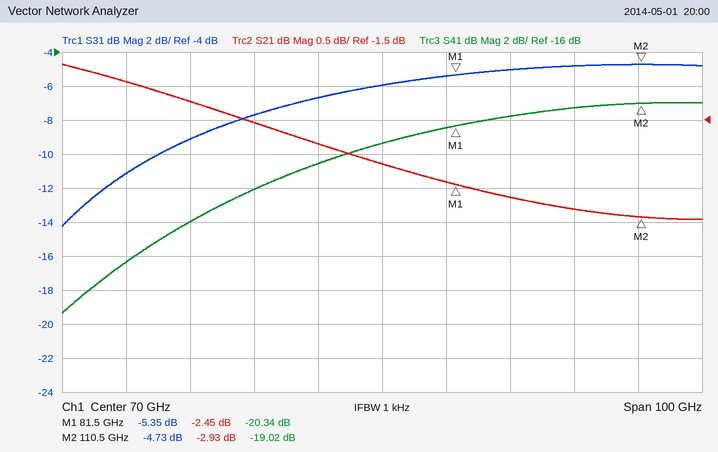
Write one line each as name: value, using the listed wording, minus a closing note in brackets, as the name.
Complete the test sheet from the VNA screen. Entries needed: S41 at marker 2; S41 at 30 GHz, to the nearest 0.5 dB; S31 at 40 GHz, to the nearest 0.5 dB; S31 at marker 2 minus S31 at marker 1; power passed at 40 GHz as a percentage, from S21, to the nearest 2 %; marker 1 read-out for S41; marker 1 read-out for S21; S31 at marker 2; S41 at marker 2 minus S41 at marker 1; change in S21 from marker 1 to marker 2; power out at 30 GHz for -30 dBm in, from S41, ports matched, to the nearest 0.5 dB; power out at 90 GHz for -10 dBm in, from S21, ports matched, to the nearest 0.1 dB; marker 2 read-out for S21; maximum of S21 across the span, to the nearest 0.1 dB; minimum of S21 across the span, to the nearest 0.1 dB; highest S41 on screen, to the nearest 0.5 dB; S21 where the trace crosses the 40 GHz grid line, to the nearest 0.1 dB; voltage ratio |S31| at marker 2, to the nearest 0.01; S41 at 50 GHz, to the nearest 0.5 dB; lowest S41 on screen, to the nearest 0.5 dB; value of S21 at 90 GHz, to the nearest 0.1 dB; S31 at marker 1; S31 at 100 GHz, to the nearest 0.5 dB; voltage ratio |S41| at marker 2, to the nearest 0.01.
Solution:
S41 at marker 2: -19.02 dB
S41 at 30 GHz, to the nearest 0.5 dB: -28.5 dB
S31 at 40 GHz, to the nearest 0.5 dB: -9.0 dB
S31 at marker 2 minus S31 at marker 1: 0.62 dB
power passed at 40 GHz as a percentage, from S21, to the nearest 2 %: 76 %
marker 1 read-out for S41: -20.34 dB
marker 1 read-out for S21: -2.45 dB
S31 at marker 2: -4.73 dB
S41 at marker 2 minus S41 at marker 1: 1.32 dB
change in S21 from marker 1 to marker 2: -0.48 dB
power out at 30 GHz for -30 dBm in, from S41, ports matched, to the nearest 0.5 dB: -58.5 dBm
power out at 90 GHz for -10 dBm in, from S21, ports matched, to the nearest 0.1 dB: -12.6 dBm
marker 2 read-out for S21: -2.93 dB
maximum of S21 across the span, to the nearest 0.1 dB: -0.7 dB
minimum of S21 across the span, to the nearest 0.1 dB: -3.0 dB
highest S41 on screen, to the nearest 0.5 dB: -19.0 dB
S21 where the trace crosses the 40 GHz grid line, to the nearest 0.1 dB: -1.2 dB
voltage ratio |S31| at marker 2, to the nearest 0.01: 0.58
S41 at 50 GHz, to the nearest 0.5 dB: -24.0 dB
lowest S41 on screen, to the nearest 0.5 dB: -31.5 dB
value of S21 at 90 GHz, to the nearest 0.1 dB: -2.6 dB
S31 at marker 1: -5.35 dB
S31 at 100 GHz, to the nearest 0.5 dB: -5.0 dB
voltage ratio |S41| at marker 2, to the nearest 0.01: 0.11
